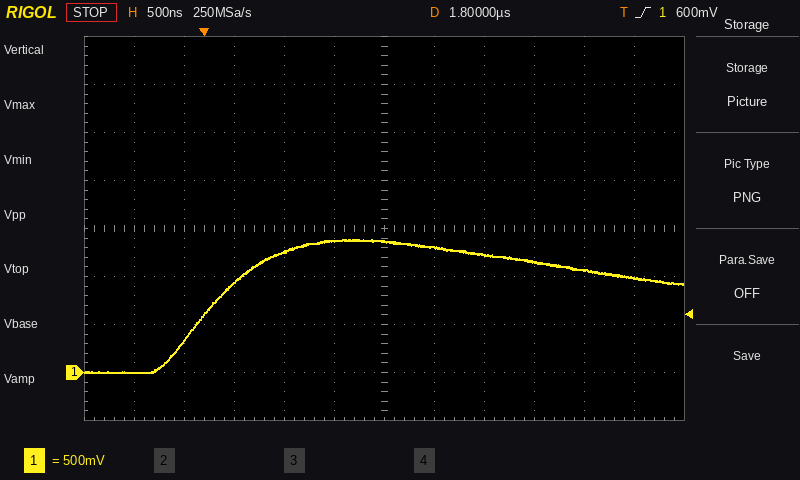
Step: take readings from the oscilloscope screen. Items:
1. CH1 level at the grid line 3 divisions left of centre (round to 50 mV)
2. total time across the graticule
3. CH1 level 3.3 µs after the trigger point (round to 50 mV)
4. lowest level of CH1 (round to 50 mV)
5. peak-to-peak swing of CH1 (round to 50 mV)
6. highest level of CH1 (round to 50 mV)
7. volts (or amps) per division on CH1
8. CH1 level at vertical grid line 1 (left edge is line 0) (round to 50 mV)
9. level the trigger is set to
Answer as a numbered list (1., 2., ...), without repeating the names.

1. 950 mV
2. 6 µs
3. 1.15 V
4. 0 mV
5. 1.40 V
6. 1.40 V
7. 500 mV
8. 0 mV
9. 600 mV
